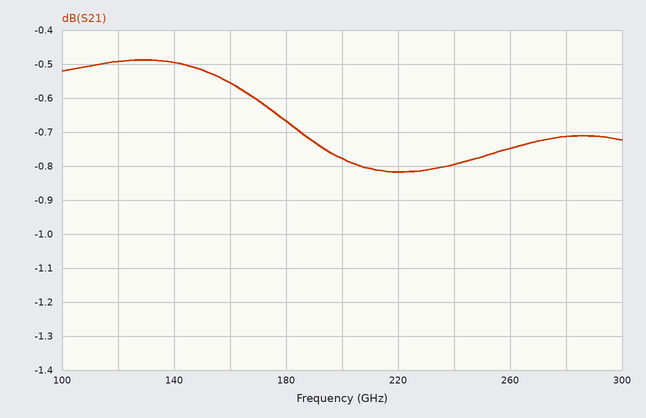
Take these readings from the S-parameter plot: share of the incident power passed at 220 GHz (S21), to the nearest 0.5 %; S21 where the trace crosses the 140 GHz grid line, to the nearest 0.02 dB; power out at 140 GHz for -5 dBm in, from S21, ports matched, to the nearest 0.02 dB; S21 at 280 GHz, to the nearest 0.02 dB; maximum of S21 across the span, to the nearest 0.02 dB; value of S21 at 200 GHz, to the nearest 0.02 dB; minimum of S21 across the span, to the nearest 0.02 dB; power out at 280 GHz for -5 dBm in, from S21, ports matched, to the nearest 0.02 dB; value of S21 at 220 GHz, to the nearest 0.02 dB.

83.0 %
-0.50 dB
-5.50 dBm
-0.72 dB
-0.48 dB
-0.78 dB
-0.82 dB
-5.72 dBm
-0.82 dB
